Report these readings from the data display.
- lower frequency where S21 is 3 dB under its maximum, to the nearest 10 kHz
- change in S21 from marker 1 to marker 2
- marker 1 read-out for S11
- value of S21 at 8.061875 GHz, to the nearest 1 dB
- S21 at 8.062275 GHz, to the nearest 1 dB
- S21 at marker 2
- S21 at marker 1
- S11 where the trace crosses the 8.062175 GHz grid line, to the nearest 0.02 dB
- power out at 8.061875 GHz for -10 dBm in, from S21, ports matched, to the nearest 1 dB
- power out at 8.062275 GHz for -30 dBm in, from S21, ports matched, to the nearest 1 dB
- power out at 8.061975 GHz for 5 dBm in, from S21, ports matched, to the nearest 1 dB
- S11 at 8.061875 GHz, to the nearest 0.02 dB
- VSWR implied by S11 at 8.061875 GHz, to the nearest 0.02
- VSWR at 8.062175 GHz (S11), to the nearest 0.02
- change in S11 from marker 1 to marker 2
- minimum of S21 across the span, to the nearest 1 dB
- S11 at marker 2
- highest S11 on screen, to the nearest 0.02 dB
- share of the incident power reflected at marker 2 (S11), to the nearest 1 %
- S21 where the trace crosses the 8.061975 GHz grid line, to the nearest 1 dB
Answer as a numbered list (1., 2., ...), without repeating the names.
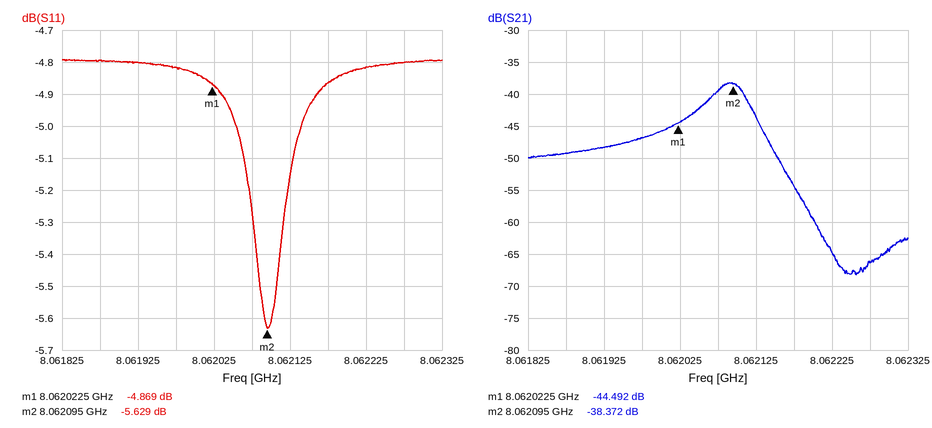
1. 8.06206 GHz
2. 6.120 dB
3. -4.869 dB
4. -49 dB
5. -66 dB
6. -38.372 dB
7. -44.492 dB
8. -4.86 dB
9. -59 dBm
10. -96 dBm
11. -42 dBm
12. -4.80 dB
13. 3.72
14. 3.66
15. -0.760 dB
16. -68 dB
17. -5.629 dB
18. -4.80 dB
19. 27 %
20. -47 dB
